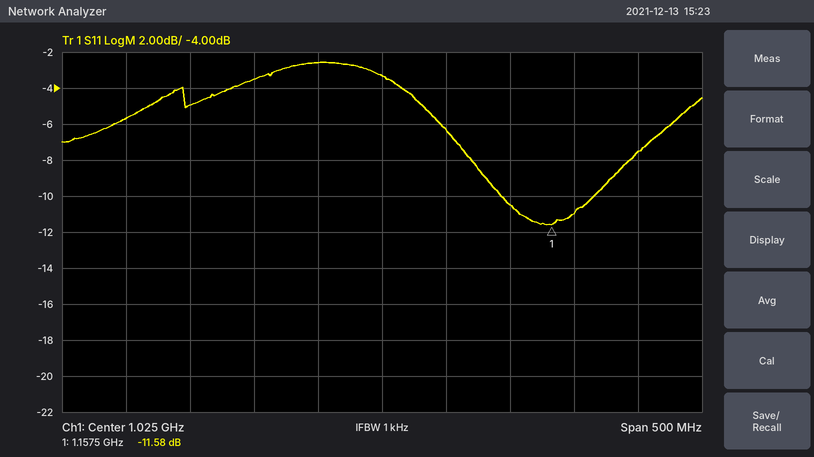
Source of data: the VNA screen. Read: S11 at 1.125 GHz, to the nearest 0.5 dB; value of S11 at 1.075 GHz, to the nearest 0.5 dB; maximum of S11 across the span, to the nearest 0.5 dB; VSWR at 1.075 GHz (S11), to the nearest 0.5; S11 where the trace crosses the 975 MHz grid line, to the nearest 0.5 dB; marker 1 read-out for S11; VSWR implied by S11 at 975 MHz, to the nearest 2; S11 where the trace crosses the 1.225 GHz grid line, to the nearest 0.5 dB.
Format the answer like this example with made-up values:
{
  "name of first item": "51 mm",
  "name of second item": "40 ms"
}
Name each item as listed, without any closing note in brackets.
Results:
{
  "S11 at 1.125 GHz, to the nearest 0.5 dB": "-10.5 dB",
  "value of S11 at 1.075 GHz, to the nearest 0.5 dB": "-6.5 dB",
  "maximum of S11 across the span, to the nearest 0.5 dB": "-2.5 dB",
  "VSWR at 1.075 GHz (S11), to the nearest 0.5": "3.0",
  "S11 where the trace crosses the 975 MHz grid line, to the nearest 0.5 dB": "-2.5 dB",
  "marker 1 read-out for S11": "-11.58 dB",
  "VSWR implied by S11 at 975 MHz, to the nearest 2": "6",
  "S11 where the trace crosses the 1.225 GHz grid line, to the nearest 0.5 dB": "-7.5 dB"
}
